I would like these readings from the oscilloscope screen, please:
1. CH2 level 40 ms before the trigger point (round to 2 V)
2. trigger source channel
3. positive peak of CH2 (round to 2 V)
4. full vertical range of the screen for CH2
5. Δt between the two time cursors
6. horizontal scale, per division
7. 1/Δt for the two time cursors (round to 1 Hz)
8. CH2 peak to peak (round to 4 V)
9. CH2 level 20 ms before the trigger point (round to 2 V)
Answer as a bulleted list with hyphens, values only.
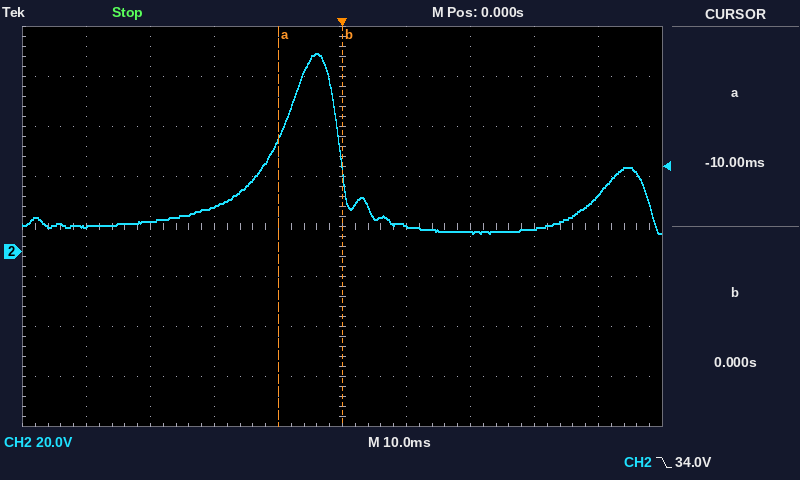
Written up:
- 10 V
- CH2
- 80 V
- 160 V
- 10 ms
- 10 ms
- 100 Hz
- 72 V
- 18 V
